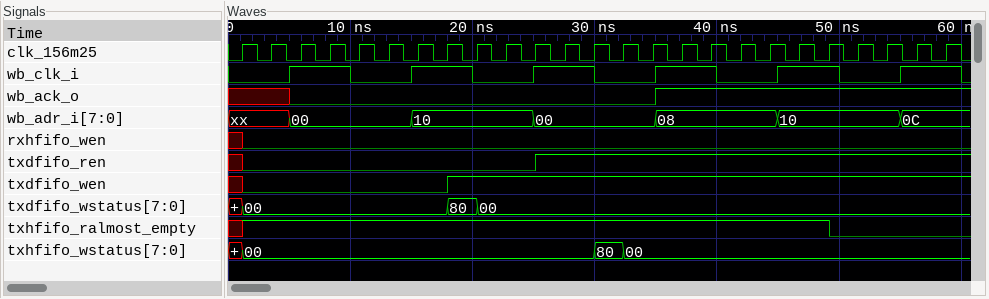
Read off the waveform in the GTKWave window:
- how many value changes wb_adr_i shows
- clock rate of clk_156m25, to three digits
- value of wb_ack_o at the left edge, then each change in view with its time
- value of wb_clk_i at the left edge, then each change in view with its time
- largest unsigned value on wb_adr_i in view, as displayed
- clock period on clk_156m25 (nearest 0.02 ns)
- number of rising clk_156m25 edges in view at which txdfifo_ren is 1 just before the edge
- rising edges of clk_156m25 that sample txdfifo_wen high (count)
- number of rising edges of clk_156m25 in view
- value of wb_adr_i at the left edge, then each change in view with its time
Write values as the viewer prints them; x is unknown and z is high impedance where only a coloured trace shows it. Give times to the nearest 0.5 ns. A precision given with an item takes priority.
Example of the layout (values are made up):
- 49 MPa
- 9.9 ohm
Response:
- 6
- 417 MHz
- x, 0 at 5 ns, 1 at 35 ns
- 0, 1 at 5 ns, 0 at 10 ns, 1 at 15 ns, 0 at 20 ns, 1 at 25 ns, 0 at 30 ns, 1 at 35 ns, 0 at 40 ns, 1 at 45 ns, 0 at 50 ns, 1 at 55 ns, 0 at 60 ns
- 10
- 2.4 ns
- 14
- 17
- 25
- xx, 00 at 5 ns, 10 at 15 ns, 00 at 25 ns, 08 at 35 ns, 10 at 45 ns, 0C at 55 ns
